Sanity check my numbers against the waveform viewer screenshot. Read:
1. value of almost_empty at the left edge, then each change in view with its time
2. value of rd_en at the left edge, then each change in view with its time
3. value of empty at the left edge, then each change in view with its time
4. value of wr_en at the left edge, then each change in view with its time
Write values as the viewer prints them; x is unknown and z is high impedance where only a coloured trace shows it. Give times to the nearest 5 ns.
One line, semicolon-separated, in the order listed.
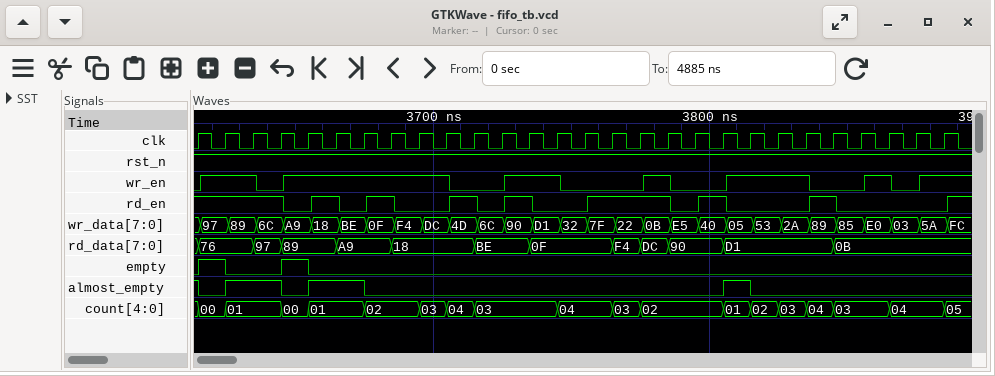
1, 0 at 3615 ns, 1 at 3625 ns, 0 at 3645 ns, 1 at 3655 ns, 0 at 3675 ns, 1 at 3805 ns, 0 at 3815 ns; 1, 0 at 3645 ns, 1 at 3655 ns, 0 at 3665 ns, 1 at 3675 ns, 0 at 3685 ns, 1 at 3705 ns, 0 at 3715 ns, 1 at 3725 ns, 0 at 3735 ns, 1 at 3755 ns, 0 at 3785 ns, 1 at 3795 ns, 0 at 3805 ns, 1 at 3835 ns, 0 at 3845 ns, 1 at 3885 ns; 0, 1 at 3615 ns, 0 at 3625 ns, 1 at 3645 ns, 0 at 3655 ns; 0, 1 at 3615 ns, 0 at 3635 ns, 1 at 3645 ns, 0 at 3705 ns, 1 at 3725 ns, 0 at 3745 ns, 1 at 3775 ns, 0 at 3785 ns, 1 at 3805 ns, 0 at 3835 ns, 1 at 3855 ns, 0 at 3865 ns, 1 at 3875 ns
